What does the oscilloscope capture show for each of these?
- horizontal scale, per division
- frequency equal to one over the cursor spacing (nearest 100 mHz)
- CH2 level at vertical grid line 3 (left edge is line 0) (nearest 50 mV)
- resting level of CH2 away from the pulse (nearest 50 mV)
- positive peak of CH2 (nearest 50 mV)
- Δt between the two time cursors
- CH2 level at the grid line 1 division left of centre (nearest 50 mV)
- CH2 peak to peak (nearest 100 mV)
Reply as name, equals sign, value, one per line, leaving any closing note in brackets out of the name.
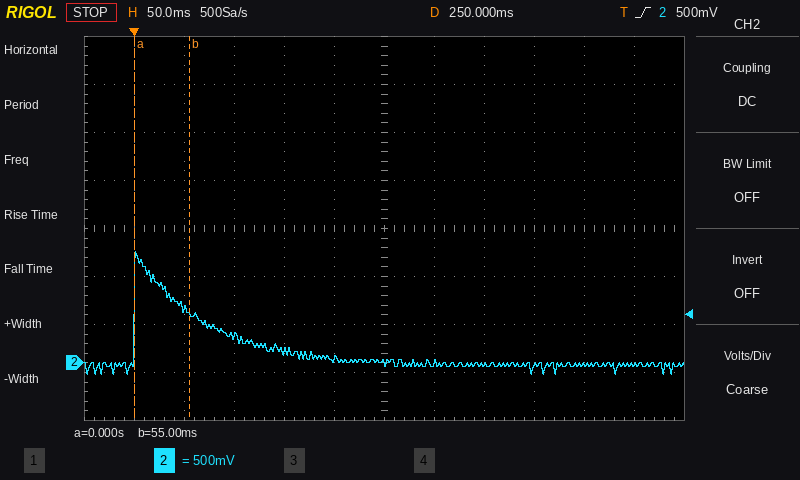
horizontal scale, per division = 50 ms
frequency equal to one over the cursor spacing = 18.2 Hz
CH2 level at vertical grid line 3 (left edge is line 0) = 300 mV
resting level of CH2 away from the pulse = 0 mV
positive peak of CH2 = 1.15 V
Δt between the two time cursors = 55 ms
CH2 level at the grid line 1 division left of centre = 50 mV
CH2 peak to peak = 1.30 V
